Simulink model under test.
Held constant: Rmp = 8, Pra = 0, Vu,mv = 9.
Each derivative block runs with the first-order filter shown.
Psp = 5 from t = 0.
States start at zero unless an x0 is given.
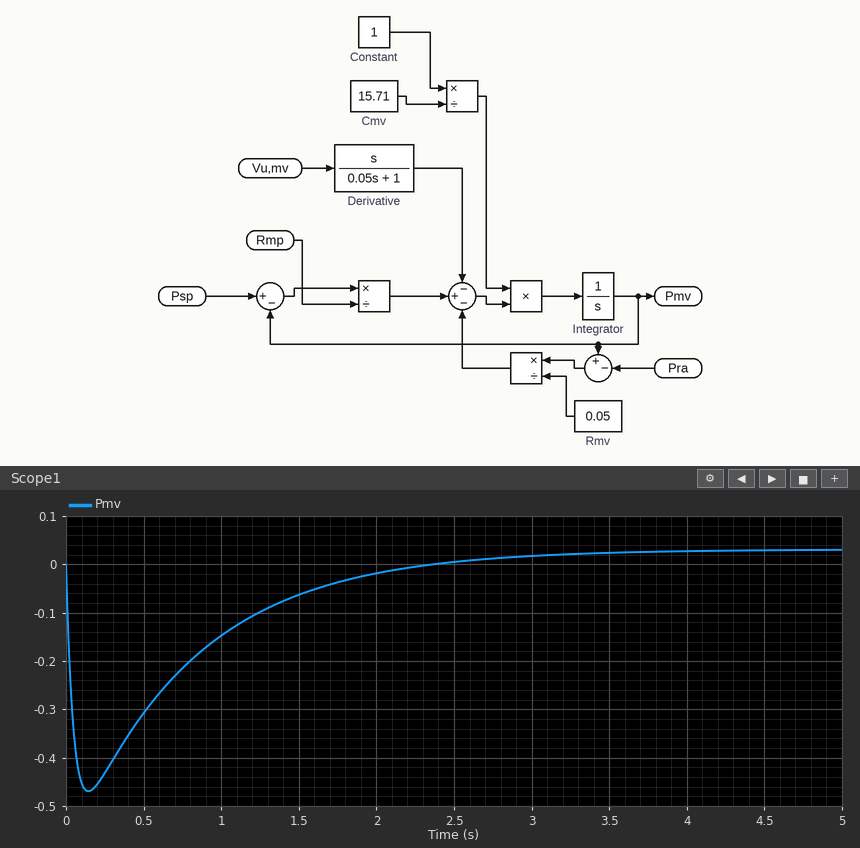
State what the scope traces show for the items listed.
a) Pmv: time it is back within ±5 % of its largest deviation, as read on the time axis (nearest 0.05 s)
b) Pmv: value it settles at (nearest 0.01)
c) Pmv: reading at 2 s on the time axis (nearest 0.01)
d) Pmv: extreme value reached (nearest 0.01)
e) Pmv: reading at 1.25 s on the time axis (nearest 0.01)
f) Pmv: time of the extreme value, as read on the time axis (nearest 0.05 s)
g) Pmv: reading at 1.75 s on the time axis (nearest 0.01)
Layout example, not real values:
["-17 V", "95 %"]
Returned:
["2.60 s", "0.03", "-0.02", "-0.47", "-0.10", "0.15 s", "-0.04"]
